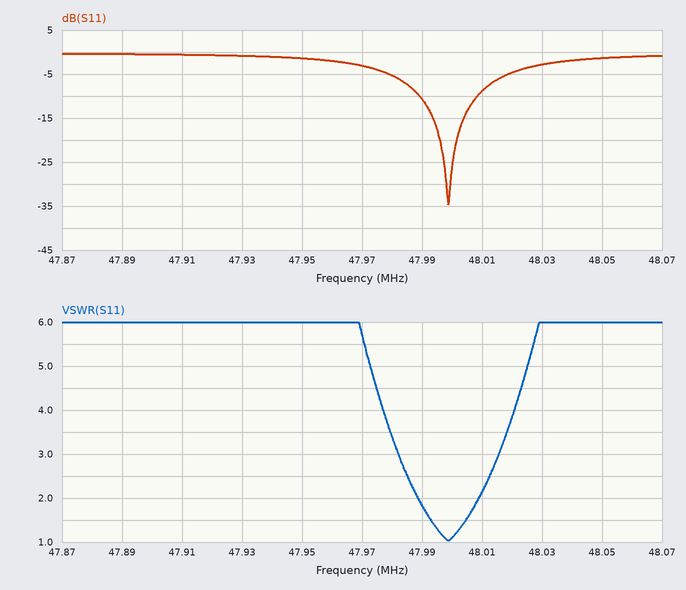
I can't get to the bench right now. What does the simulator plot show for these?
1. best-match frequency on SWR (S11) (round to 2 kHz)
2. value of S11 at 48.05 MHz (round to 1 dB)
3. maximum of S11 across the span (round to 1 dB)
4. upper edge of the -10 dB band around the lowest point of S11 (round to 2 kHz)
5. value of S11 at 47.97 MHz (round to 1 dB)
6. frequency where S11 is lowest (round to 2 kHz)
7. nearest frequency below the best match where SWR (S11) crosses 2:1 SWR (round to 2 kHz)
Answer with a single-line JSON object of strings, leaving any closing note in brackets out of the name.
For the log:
{"best-match frequency on SWR (S11)": "47.998 MHz", "value of S11 at 48.05 MHz": "-1 dB", "maximum of S11 across the span": "0 dB", "upper edge of the -10 dB band around the lowest point of S11": "48.008 MHz", "value of S11 at 47.97 MHz": "-3 dB", "frequency where S11 is lowest": "47.998 MHz", "nearest frequency below the best match where SWR (S11) crosses 2:1 SWR": "47.988 MHz"}
